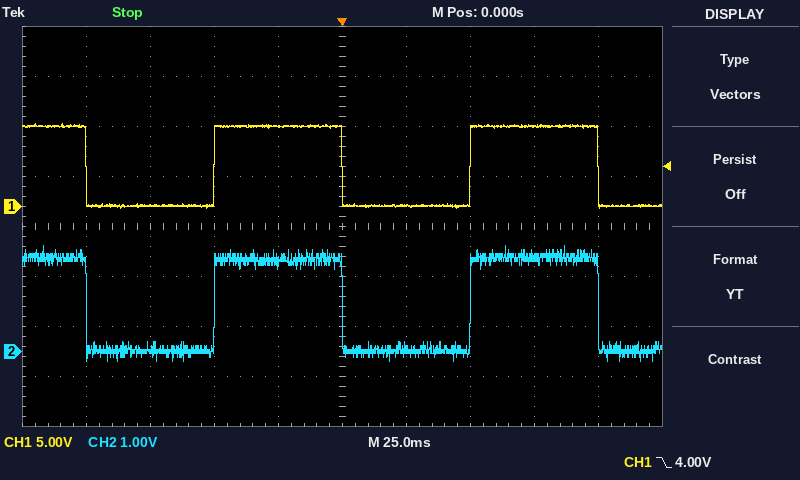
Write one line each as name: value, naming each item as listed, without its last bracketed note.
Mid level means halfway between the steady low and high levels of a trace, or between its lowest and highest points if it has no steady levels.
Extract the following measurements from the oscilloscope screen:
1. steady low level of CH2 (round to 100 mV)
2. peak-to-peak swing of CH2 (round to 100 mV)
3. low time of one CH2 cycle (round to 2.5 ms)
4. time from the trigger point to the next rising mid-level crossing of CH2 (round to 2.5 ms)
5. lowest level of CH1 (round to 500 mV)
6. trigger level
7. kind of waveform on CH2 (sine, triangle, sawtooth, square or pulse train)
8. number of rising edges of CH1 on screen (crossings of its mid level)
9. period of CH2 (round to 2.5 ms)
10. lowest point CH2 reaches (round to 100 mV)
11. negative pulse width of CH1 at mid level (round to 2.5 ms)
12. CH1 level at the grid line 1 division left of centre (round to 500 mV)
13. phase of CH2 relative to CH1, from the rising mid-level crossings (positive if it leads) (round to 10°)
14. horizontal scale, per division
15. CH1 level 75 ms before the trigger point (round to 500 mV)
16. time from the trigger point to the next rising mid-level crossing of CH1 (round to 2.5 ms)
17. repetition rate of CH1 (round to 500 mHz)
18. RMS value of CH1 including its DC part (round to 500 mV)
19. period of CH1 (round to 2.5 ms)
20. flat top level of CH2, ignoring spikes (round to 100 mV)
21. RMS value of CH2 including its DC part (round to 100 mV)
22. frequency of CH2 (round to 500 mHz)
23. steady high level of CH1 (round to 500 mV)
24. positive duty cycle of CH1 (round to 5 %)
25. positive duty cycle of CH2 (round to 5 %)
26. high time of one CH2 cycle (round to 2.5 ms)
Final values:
steady low level of CH2: 0.0 V
peak-to-peak swing of CH2: 2.3 V
low time of one CH2 cycle: 50.0 ms
time from the trigger point to the next rising mid-level crossing of CH2: 50.0 ms
lowest level of CH1: 0.0 V
trigger level: 4.00 V
kind of waveform on CH2: square
number of rising edges of CH1 on screen: 2
period of CH2: 100.0 ms
lowest point CH2 reaches: -200 mV
negative pulse width of CH1 at mid level: 50.0 ms
CH1 level at the grid line 1 division left of centre: 8.0 V
phase of CH2 relative to CH1, from the rising mid-level crossings (positive if it leads): 0°
horizontal scale, per division: 25 ms
CH1 level 75 ms before the trigger point: 0.0 V
time from the trigger point to the next rising mid-level crossing of CH1: 50.0 ms
repetition rate of CH1: 10.0 Hz
RMS value of CH1 including its DC part: 5.5 V
period of CH1: 100.0 ms
flat top level of CH2, ignoring spikes: 1.9 V
RMS value of CH2 including its DC part: 1.3 V
frequency of CH2: 10.0 Hz
steady high level of CH1: 8.0 V
positive duty cycle of CH1: 50 %
positive duty cycle of CH2: 50 %
high time of one CH2 cycle: 50.0 ms
